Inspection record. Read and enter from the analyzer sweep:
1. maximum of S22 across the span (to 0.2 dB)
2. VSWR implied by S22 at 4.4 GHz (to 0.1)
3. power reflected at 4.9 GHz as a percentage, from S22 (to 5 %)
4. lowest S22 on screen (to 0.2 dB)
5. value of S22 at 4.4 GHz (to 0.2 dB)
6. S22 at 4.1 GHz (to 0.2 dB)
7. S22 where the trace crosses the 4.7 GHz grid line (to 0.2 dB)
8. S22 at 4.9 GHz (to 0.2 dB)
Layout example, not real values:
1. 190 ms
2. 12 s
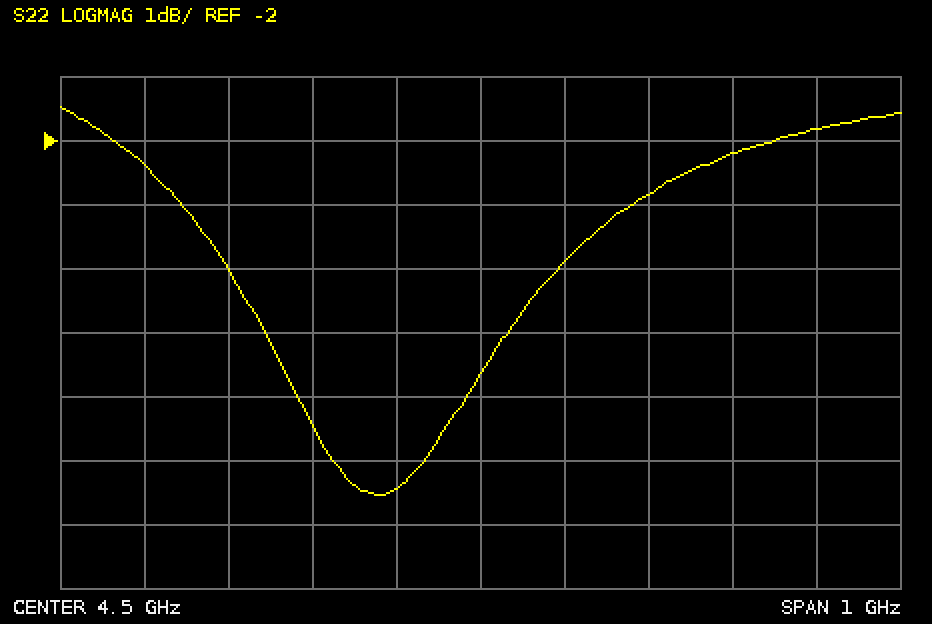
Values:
1. -1.4 dB
2. 2.5
3. 65 %
4. -7.6 dB
5. -7.4 dB
6. -2.4 dB
7. -2.8 dB
8. -1.8 dB
